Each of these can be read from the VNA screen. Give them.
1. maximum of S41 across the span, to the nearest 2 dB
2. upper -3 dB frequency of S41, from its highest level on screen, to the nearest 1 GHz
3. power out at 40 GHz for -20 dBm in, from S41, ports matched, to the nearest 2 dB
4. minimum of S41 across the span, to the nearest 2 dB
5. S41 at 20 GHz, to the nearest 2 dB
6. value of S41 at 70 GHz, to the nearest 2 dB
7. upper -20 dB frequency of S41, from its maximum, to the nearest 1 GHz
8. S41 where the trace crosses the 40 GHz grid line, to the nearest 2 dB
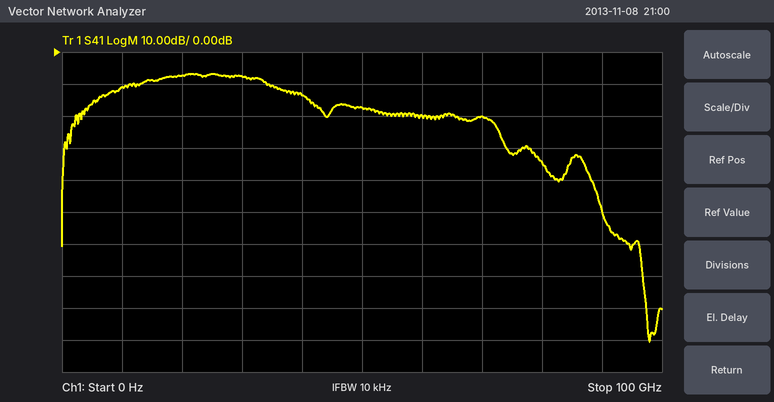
-6 dB
34 GHz
-34 dBm
-90 dB
-8 dB
-20 dB
73 GHz
-14 dB
